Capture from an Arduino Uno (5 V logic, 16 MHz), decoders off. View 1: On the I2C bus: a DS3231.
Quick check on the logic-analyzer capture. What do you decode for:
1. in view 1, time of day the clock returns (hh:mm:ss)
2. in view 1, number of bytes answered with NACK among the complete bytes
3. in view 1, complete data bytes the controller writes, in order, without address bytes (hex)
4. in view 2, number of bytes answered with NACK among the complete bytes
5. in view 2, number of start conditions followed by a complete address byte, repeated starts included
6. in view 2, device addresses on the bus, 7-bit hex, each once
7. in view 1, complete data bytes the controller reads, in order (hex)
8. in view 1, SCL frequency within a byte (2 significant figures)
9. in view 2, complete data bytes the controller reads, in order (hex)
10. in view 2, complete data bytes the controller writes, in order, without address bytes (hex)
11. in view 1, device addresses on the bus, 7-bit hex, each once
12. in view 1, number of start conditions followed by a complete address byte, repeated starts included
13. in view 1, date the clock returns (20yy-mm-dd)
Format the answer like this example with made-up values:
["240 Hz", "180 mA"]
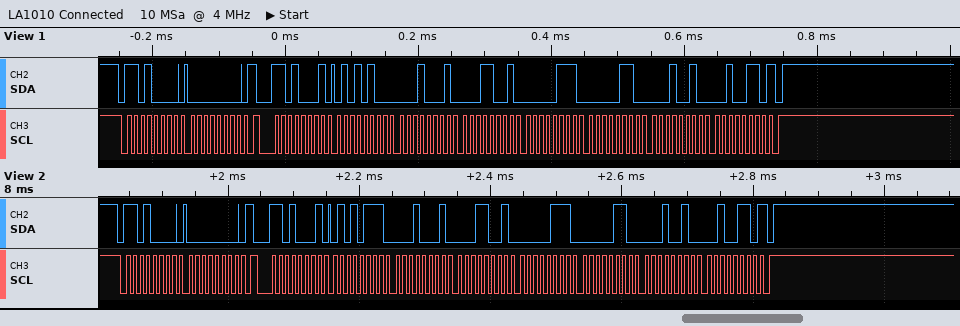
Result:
["19:11:54", "1", "00", "1", "2", "0x68", "54 11 19 07 06 12 26", "100 kHz", "57 11 19 07 06 12 26", "00", "0x68", "2", "2026-12-06"]
